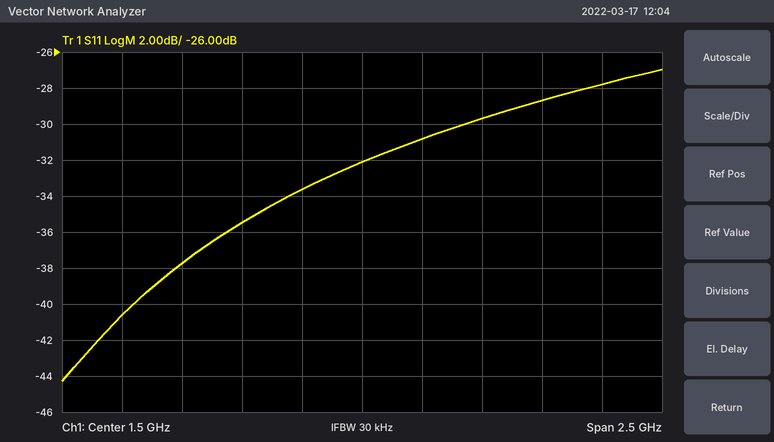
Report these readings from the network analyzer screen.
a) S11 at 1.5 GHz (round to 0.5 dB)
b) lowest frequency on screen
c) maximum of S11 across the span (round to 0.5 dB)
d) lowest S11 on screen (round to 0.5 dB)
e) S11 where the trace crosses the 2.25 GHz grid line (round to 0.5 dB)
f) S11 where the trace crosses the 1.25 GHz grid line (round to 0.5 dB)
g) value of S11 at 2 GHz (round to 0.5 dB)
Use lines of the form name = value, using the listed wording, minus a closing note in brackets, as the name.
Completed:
S11 at 1.5 GHz = -32.0 dB
lowest frequency on screen = 250 MHz
maximum of S11 across the span = -27.0 dB
lowest S11 on screen = -44.5 dB
S11 where the trace crosses the 2.25 GHz grid line = -28.5 dB
S11 where the trace crosses the 1.25 GHz grid line = -33.5 dB
value of S11 at 2 GHz = -29.5 dB
